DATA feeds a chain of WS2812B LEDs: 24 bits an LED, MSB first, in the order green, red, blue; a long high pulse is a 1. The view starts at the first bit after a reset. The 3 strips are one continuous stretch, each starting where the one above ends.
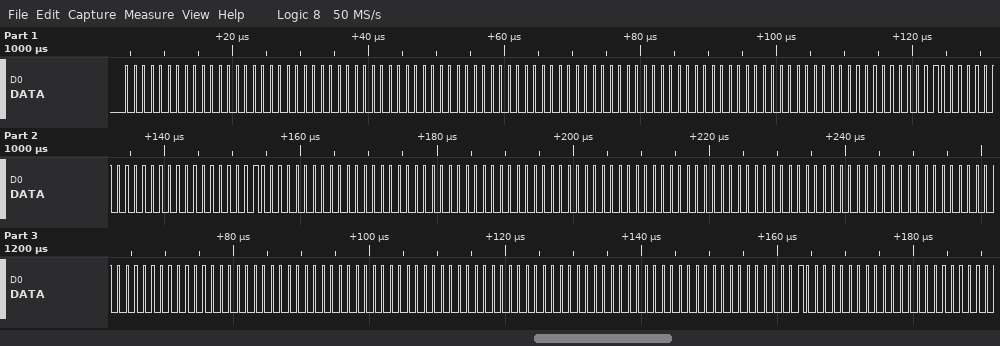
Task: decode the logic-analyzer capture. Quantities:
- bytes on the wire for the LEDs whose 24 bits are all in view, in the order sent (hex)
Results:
00 00 00 00 00 00 00 00 00 00 00 01 00 00 01 00 00 00 00 00 00 00 00 00 00 00 00 00 00 00 00 00 00 00 00 01
